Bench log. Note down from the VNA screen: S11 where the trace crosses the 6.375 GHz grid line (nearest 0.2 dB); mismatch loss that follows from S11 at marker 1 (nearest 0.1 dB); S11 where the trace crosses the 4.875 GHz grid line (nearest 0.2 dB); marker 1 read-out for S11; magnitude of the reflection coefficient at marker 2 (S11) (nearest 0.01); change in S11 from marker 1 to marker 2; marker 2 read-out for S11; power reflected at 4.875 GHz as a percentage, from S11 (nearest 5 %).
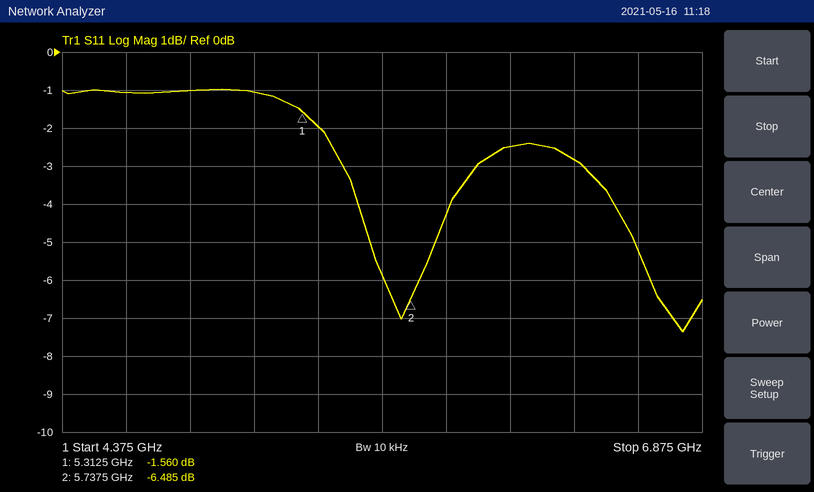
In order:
-2.8 dB
5.2 dB
-1.0 dB
-1.560 dB
0.47
-4.925 dB
-6.485 dB
80 %
